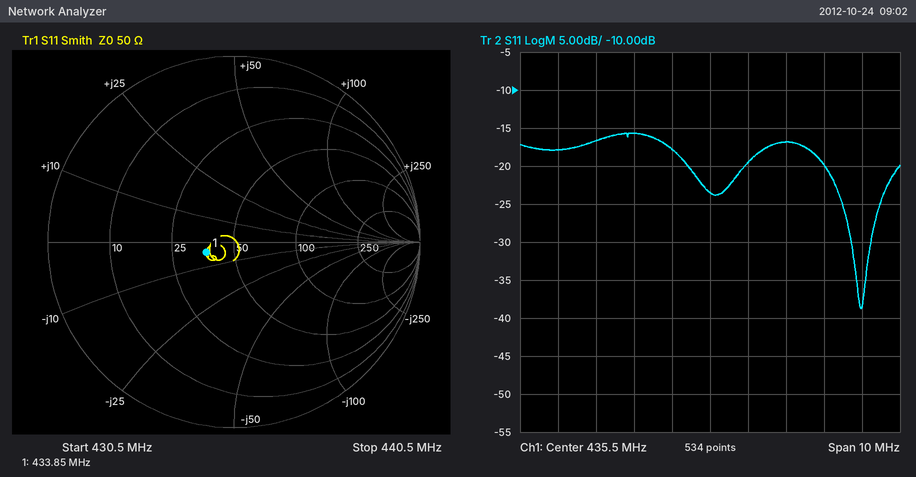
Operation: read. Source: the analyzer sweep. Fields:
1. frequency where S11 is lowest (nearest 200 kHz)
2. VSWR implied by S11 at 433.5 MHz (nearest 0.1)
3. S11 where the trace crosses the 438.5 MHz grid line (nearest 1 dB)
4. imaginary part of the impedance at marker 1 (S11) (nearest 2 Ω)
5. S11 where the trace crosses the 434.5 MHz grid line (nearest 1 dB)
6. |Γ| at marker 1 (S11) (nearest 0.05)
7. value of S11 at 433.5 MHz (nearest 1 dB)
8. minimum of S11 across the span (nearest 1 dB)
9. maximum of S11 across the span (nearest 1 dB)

439.4 MHz
1.4
-20 dB
-4 Ω
-18 dB
0.15
-16 dB
-39 dB
-16 dB
